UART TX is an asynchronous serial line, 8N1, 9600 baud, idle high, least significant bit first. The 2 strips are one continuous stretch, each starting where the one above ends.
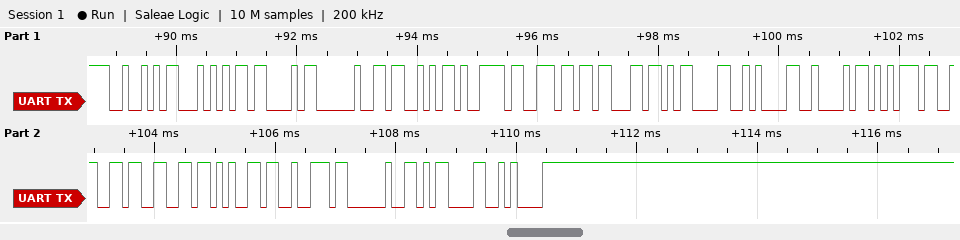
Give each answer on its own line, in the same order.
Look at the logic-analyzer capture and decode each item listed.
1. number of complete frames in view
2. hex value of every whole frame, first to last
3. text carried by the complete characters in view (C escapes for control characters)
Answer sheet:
19
52 54 43 20 53 79 6E 63 0D 0A 42 75 66 66 65 72 20 0D 0A
"RTC Sync\r\nBuffer \r\n"
